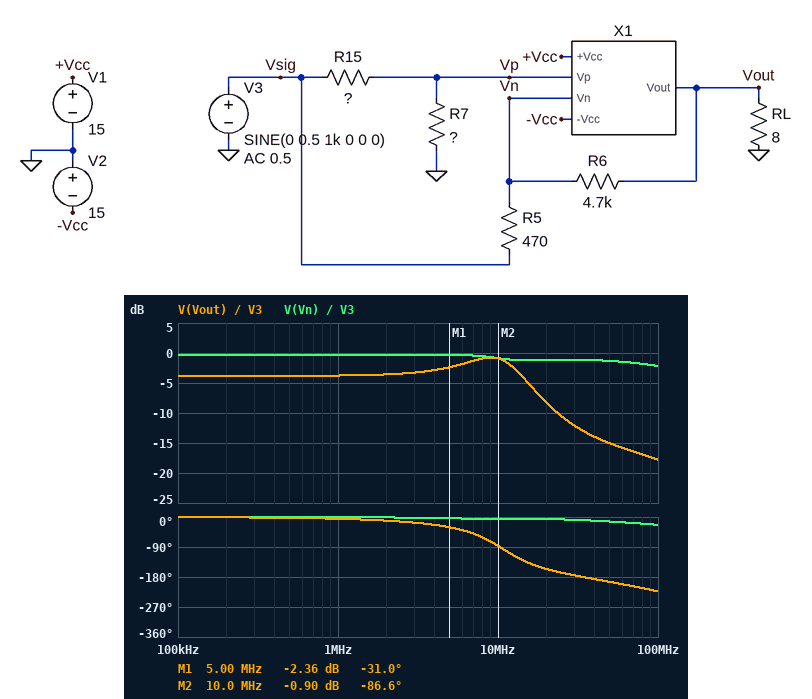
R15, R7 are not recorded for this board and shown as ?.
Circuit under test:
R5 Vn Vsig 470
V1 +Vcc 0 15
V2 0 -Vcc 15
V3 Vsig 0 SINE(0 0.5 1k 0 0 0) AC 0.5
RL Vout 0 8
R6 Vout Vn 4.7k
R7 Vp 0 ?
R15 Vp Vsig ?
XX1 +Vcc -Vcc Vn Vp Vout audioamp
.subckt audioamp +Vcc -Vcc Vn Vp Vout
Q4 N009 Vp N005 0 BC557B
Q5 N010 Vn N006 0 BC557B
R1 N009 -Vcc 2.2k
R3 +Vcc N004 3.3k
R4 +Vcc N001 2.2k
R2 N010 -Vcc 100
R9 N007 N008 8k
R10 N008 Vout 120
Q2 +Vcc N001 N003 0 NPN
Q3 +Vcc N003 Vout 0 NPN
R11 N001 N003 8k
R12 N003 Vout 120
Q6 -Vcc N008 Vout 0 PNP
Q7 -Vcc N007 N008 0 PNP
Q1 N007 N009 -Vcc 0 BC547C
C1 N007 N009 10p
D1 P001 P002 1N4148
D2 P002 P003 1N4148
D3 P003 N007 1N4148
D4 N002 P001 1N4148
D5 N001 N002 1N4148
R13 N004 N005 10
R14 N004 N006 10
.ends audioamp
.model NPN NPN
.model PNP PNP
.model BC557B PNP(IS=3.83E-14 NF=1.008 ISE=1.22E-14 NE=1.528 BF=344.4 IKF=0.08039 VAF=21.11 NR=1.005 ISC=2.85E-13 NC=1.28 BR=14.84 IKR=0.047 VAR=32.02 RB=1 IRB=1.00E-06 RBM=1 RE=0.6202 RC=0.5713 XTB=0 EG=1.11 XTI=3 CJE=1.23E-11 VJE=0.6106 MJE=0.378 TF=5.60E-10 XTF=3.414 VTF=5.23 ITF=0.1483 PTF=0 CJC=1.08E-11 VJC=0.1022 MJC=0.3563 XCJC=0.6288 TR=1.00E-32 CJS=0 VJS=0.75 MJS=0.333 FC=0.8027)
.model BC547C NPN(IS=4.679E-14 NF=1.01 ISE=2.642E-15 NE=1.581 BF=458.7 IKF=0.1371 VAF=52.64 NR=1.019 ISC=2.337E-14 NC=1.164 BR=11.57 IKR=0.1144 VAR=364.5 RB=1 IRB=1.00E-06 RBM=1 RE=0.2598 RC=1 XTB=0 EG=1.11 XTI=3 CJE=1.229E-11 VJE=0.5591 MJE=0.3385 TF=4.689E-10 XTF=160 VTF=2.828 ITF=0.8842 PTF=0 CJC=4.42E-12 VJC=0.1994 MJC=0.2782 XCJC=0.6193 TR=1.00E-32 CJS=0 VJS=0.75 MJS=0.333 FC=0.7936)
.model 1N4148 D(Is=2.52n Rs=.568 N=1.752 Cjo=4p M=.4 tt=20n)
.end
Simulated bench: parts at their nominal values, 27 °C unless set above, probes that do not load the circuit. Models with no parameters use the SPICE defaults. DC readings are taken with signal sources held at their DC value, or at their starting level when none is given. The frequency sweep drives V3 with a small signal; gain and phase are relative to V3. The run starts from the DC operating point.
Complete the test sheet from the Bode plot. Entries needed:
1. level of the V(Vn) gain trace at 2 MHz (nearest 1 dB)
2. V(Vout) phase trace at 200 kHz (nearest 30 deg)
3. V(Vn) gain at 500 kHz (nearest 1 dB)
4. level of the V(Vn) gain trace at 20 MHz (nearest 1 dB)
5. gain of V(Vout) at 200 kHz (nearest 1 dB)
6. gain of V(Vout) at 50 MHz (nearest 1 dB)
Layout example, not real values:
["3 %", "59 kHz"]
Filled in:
["0 dB", "0 deg", "0 dB", "-1 dB", "-4 dB", "-15 dB"]
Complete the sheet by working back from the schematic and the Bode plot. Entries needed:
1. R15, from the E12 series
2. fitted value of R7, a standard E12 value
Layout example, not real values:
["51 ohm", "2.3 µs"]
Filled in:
["390 Ω", "10 kΩ"]
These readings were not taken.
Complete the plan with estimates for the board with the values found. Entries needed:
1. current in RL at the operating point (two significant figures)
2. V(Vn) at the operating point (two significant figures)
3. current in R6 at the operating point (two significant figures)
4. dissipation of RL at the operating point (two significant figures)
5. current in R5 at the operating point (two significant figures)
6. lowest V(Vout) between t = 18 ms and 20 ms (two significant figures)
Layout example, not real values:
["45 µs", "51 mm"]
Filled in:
["150 mA", "-110 mV", "230 µA", "180 mW", "230 µA", "-1.5 V"]
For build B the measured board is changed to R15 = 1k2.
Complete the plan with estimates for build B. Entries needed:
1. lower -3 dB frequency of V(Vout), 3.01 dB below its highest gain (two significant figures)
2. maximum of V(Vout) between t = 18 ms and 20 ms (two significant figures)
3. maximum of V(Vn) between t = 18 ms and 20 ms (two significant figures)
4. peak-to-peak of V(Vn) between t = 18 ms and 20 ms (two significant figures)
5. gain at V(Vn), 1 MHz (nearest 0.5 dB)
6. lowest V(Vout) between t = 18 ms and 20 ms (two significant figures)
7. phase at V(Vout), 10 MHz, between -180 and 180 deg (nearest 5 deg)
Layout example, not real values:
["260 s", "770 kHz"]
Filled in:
["5.0 MHz", "-1.1 V", "340 mV", "900 mV", "-1.0 dB", "-1.3 V", "135 deg"]
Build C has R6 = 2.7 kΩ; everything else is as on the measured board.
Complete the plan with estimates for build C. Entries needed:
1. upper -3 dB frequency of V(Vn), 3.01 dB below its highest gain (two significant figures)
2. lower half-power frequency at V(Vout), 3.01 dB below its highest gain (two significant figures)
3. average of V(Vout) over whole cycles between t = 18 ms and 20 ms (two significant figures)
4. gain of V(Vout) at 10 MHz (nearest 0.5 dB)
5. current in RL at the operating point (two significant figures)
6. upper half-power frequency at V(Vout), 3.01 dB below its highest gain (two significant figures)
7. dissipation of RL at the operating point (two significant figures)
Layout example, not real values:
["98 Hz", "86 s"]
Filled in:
["150 MHz", "6.6 MHz", "-740 mV", "2.0 dB", "92 mA", "17 MHz", "68 mW"]
